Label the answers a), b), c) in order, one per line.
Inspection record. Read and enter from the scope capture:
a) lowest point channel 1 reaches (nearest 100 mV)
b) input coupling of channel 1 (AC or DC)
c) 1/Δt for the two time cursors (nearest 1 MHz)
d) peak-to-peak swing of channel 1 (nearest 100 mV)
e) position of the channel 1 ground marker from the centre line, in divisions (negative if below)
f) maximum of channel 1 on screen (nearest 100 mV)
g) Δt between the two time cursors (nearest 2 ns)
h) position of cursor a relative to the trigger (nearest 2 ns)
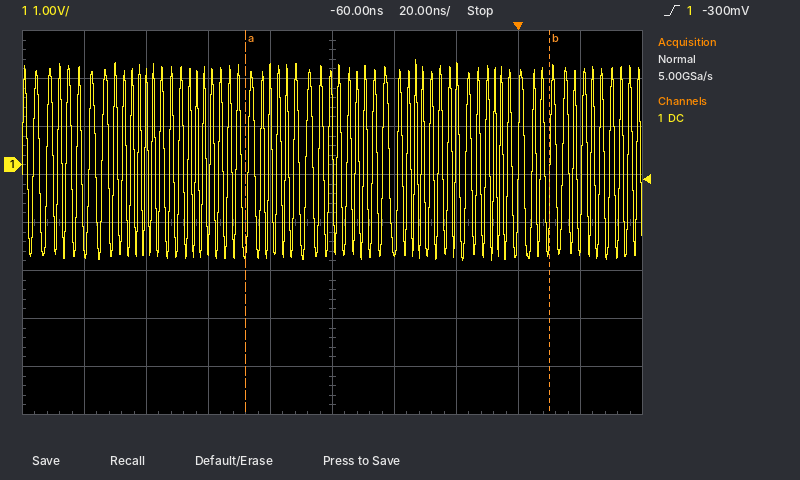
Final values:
a) -2.0 V
b) DC
c) 10 MHz
d) 4.2 V
e) +1.2 div
f) 2.2 V
g) 98 ns
h) -88 ns
